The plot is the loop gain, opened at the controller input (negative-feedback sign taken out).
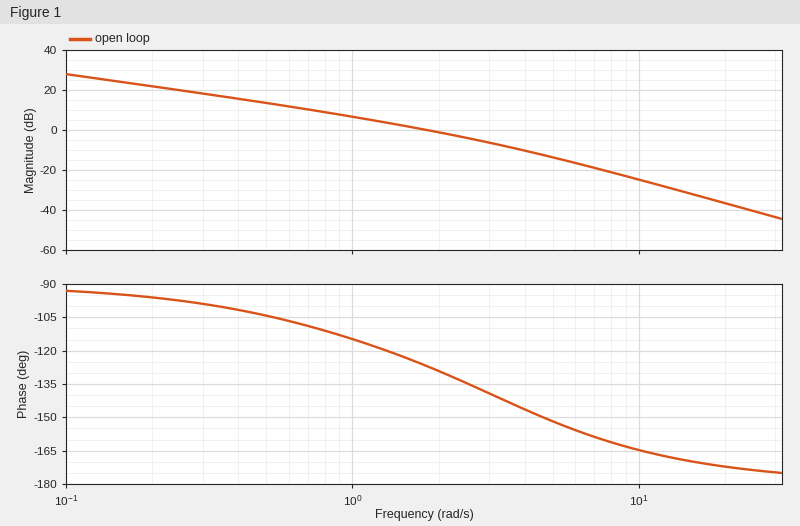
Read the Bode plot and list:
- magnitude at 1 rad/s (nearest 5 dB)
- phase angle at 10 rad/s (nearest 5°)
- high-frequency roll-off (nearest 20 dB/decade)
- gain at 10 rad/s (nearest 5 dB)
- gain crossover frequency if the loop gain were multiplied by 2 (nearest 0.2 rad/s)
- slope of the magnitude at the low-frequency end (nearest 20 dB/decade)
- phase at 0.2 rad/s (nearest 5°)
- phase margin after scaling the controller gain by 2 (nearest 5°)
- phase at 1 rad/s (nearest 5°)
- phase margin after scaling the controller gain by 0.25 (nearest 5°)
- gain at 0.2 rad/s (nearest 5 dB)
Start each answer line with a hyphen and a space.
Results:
- 5 dB
- -165°
- -40 dB/decade
- -25 dB
- 3.0 rad/s
- -20 dB/decade
- -95°
- 40°
- -115°
- 75°
- 20 dB
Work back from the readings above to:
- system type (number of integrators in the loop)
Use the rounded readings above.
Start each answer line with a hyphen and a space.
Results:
- 1
